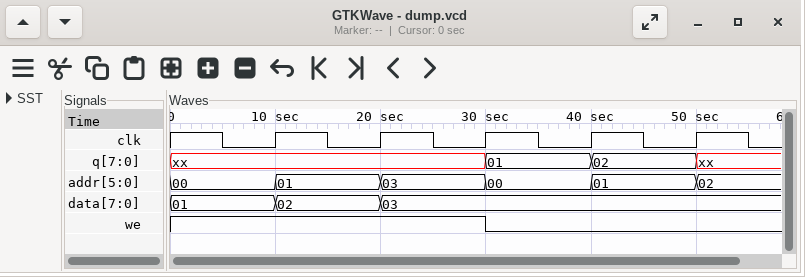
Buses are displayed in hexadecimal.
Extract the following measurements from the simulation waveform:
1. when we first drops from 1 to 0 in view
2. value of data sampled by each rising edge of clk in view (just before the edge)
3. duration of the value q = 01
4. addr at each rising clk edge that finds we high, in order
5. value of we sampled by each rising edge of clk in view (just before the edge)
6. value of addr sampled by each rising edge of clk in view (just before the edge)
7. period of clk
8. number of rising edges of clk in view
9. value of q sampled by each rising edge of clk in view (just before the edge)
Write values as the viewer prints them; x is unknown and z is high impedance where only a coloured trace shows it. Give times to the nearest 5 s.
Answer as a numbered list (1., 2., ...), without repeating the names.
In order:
1. 30 s
2. 01, 02, 03, 03, 03
3. 10 s
4. 00, 01, 03
5. 1 1 1 0 0
6. 00, 01, 03, 00, 01
7. 10 s
8. 5
9. xx, xx, xx, 01, 02
